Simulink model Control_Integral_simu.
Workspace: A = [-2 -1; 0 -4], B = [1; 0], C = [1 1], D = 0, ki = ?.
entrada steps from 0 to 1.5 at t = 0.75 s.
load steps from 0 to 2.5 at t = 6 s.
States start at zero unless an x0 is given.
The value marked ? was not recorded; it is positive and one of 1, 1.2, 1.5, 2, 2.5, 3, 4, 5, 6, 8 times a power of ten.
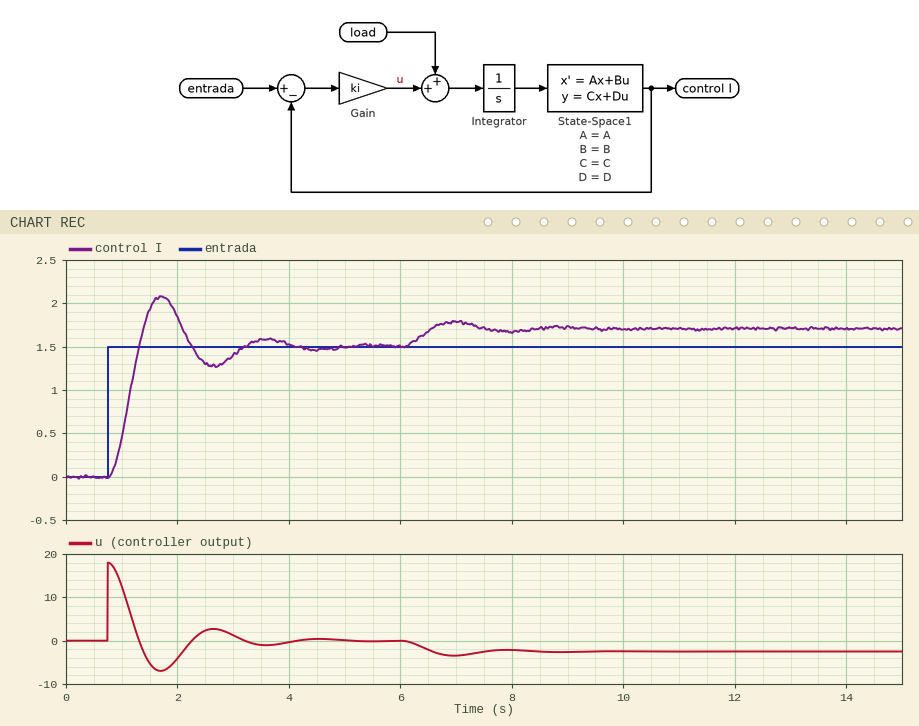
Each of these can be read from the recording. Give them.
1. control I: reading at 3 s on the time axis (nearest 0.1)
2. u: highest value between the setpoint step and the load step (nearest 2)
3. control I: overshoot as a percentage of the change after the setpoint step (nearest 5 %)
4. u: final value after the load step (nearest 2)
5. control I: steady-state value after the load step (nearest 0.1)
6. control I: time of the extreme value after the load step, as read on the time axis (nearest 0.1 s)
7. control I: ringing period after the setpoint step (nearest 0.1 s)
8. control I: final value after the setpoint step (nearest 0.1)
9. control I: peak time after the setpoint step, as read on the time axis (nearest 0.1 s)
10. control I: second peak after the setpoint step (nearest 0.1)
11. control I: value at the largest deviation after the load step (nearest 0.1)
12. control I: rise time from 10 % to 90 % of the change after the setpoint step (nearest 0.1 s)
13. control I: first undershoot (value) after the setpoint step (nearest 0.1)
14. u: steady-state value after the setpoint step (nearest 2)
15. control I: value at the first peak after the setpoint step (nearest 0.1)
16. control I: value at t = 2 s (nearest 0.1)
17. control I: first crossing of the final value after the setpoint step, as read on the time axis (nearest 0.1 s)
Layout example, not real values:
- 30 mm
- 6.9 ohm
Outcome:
- 1.4
- 18
- 40 %
- -2
- 1.7
- 7.0 s
- 1.9 s
- 1.5
- 1.7 s
- 1.6
- 1.8
- 0.4 s
- 1.3
- 0
- 2.1
- 1.8
- 1.3 s
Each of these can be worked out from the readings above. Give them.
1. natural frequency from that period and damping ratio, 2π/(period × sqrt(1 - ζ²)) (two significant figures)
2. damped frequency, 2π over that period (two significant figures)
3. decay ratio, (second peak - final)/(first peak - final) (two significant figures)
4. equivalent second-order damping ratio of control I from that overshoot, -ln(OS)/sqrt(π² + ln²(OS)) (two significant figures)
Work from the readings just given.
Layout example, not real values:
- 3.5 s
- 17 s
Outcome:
- 3.4 rad/s
- 3.3 rad/s
- 0.17
- 0.28
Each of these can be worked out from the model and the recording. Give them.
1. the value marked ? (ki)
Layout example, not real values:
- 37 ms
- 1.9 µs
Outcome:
- 12
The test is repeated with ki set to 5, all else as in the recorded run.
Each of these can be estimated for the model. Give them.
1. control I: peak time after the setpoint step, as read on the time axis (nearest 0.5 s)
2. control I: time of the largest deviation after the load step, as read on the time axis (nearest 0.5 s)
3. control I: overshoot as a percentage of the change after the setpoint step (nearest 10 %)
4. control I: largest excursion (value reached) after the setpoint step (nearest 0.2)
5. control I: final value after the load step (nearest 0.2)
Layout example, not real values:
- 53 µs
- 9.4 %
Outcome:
- 2.5 s
- 7.5 s
- 20 %
- 1.8
- 2.0
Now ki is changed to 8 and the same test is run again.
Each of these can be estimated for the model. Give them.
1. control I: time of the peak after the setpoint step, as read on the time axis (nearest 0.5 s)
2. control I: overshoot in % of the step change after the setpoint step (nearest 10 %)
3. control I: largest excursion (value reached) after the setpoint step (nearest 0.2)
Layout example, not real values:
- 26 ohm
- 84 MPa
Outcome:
- 2.0 s
- 30 %
- 2.0
